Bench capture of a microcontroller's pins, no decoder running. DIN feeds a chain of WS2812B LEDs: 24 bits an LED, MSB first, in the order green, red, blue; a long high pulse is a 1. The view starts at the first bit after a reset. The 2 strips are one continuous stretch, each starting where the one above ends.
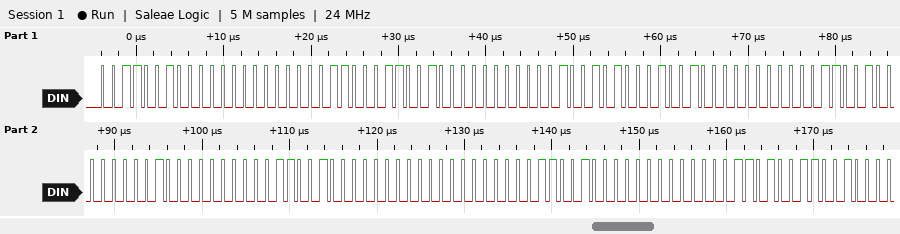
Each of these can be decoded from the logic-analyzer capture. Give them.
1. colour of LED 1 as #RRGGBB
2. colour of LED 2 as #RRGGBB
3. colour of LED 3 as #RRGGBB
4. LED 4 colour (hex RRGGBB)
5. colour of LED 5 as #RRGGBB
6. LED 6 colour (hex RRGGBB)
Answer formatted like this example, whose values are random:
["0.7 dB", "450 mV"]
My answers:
["#003206", "#003225", "#001232", "#000132", "#000032", "#0D0032"]
